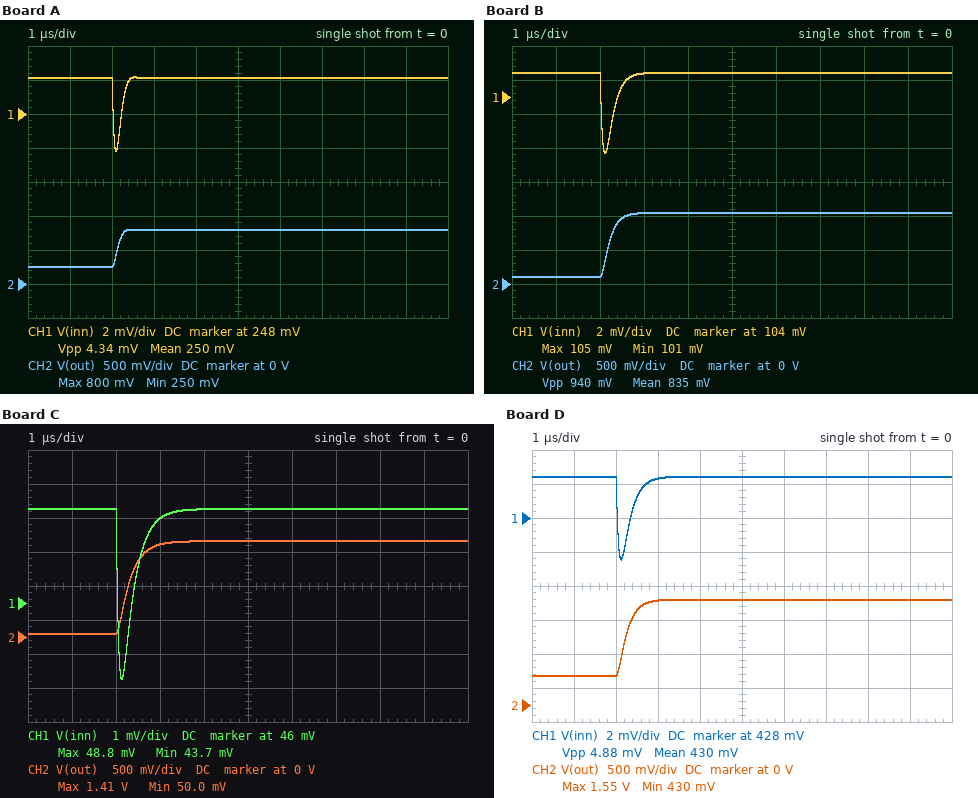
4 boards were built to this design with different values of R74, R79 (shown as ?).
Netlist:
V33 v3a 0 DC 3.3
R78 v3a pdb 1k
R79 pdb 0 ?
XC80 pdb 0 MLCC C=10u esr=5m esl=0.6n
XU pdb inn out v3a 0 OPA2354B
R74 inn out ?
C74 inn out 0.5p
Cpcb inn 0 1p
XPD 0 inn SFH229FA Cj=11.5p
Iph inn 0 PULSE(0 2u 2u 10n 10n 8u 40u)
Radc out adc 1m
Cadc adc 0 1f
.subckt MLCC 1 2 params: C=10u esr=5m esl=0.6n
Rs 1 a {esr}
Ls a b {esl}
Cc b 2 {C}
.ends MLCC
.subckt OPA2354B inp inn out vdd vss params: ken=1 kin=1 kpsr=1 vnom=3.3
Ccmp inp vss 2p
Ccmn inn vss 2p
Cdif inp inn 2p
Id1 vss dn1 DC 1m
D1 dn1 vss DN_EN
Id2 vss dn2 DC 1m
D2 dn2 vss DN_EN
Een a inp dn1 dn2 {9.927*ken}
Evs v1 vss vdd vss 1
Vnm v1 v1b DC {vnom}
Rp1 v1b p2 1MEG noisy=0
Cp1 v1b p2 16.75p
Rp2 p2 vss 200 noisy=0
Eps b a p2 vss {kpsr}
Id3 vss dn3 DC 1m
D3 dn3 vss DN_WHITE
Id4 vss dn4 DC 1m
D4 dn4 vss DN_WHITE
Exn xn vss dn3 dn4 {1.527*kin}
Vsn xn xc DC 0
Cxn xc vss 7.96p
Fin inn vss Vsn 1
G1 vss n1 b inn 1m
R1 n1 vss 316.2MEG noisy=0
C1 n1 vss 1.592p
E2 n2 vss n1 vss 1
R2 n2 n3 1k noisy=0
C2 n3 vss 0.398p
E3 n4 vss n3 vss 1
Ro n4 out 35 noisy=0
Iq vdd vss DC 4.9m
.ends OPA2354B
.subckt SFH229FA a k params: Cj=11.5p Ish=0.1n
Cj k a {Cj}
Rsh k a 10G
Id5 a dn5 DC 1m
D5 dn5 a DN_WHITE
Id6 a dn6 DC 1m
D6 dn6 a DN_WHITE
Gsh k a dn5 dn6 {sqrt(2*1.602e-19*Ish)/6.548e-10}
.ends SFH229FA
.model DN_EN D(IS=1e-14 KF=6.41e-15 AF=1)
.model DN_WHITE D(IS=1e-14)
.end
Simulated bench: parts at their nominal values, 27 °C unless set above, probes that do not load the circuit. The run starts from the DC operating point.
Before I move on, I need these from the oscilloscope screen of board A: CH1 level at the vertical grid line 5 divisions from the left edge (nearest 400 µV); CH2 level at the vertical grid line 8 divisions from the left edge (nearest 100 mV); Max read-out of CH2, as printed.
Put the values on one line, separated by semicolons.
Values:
250.0 mV; 800 mV; 800 mV
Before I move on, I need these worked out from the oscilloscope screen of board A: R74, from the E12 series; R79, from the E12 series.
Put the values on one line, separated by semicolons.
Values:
270 kΩ; 82 Ω
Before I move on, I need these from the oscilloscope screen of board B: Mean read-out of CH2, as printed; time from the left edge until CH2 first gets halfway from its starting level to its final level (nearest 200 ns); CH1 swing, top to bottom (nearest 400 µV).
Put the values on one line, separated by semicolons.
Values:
835 mV; 2.2 µs; 4.8 mV
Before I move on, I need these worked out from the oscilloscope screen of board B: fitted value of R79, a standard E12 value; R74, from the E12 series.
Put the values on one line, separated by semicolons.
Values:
33 Ω; 470 kΩ
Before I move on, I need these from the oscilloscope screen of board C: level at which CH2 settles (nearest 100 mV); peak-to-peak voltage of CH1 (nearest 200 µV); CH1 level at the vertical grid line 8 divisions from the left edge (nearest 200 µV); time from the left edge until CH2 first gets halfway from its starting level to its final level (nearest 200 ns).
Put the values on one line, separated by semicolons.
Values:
1.4 V; 5.0 mV; 48.8 mV; 2.2 µs
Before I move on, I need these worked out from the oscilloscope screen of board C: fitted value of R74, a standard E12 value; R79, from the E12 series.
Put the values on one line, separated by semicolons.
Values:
680 kΩ; 15 Ω
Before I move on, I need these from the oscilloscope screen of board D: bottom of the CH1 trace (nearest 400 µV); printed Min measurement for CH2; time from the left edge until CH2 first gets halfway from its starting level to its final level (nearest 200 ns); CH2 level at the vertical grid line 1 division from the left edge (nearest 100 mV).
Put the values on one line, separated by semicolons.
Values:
425.6 mV; 430 mV; 2.2 µs; 400 mV
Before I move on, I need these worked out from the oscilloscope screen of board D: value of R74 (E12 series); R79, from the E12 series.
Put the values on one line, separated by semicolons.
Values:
560 kΩ; 150 Ω
